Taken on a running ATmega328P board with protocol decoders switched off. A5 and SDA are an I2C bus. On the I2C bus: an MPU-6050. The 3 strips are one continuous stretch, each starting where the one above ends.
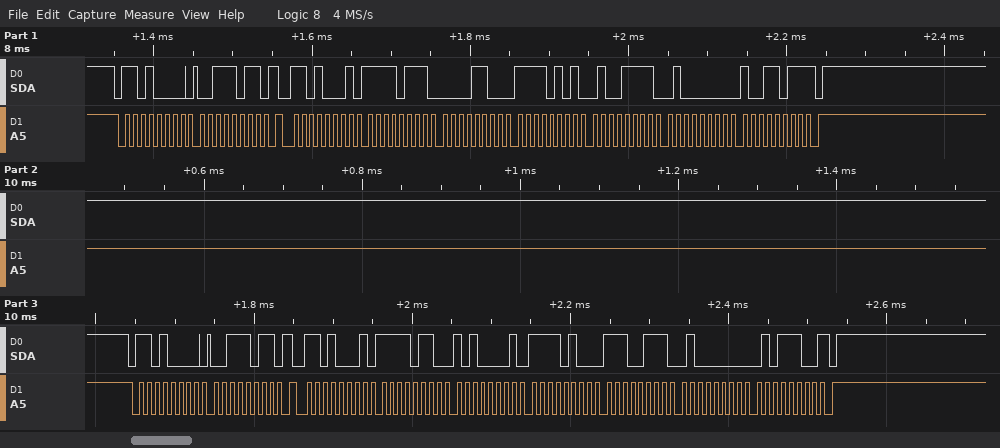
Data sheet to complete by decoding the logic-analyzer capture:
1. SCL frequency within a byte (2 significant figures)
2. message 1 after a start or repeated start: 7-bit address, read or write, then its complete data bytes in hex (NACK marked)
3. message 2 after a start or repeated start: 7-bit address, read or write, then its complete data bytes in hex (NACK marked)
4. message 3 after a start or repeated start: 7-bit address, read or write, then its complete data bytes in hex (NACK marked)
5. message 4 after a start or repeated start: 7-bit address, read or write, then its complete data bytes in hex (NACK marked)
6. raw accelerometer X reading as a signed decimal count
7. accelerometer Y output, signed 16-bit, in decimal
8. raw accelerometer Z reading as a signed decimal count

100 kHz
0x68 write: 3B
0x68 read: F7 0C F5 4F 40 9B NACK
0x68 write: 3B
0x68 read: F6 A1 F4 E7 40 5C NACK
-2292
-2737
16539
